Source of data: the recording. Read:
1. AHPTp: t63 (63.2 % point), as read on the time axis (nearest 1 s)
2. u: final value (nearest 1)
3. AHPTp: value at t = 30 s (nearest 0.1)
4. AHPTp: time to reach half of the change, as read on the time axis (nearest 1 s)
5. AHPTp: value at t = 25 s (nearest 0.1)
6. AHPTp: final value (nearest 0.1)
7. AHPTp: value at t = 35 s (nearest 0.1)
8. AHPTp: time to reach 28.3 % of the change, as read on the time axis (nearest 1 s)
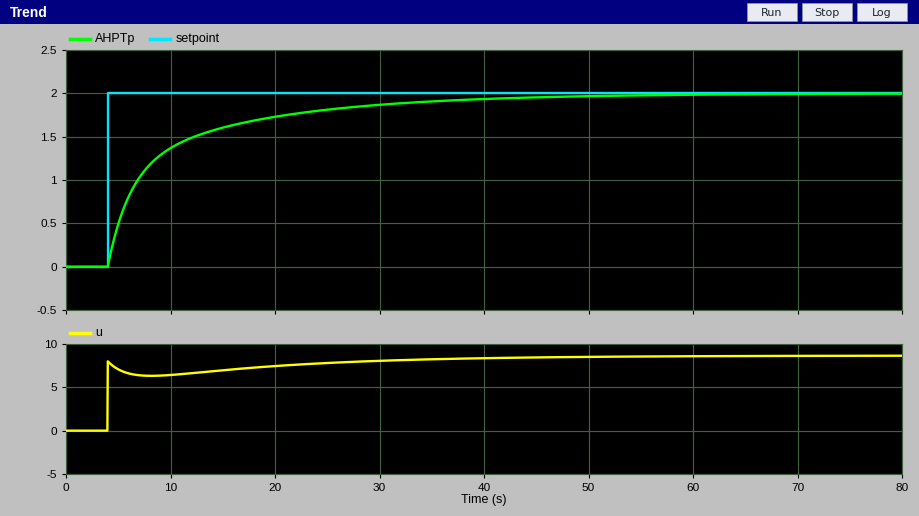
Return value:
9 s
9
1.9
7 s
1.8
2.0
1.9
5 s
